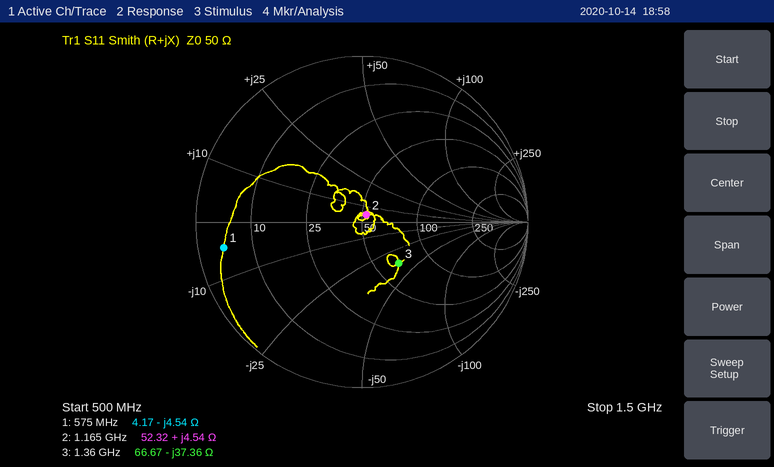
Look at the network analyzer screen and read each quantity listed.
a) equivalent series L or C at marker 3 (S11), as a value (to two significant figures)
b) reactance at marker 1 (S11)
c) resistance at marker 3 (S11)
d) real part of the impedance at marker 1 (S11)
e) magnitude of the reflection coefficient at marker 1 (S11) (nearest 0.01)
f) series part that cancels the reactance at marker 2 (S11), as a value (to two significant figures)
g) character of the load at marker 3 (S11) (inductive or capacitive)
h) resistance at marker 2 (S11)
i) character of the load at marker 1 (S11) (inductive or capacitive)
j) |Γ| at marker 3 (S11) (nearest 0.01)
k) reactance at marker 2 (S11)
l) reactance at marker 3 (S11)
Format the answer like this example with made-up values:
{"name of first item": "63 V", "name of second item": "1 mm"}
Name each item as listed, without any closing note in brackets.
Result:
{"equivalent series L or C at marker 3 (S11), as a value": "3.1 pF", "reactance at marker 1": "-4.54 Ω", "resistance at marker 3": "66.67 Ω", "real part of the impedance at marker 1": "4.17 Ω", "magnitude of the reflection coefficient at marker 1 (S11)": "0.85", "series part that cancels the reactance at marker 2 (S11), as a value": "30 pF", "character of the load at marker 3 (S11)": "capacitive", "resistance at marker 2": "52.32 Ω", "character of the load at marker 1 (S11)": "capacitive", "|Γ| at marker 3 (S11)": "0.33", "reactance at marker 2": "+4.54 Ω", "reactance at marker 3": "-37.36 Ω"}
